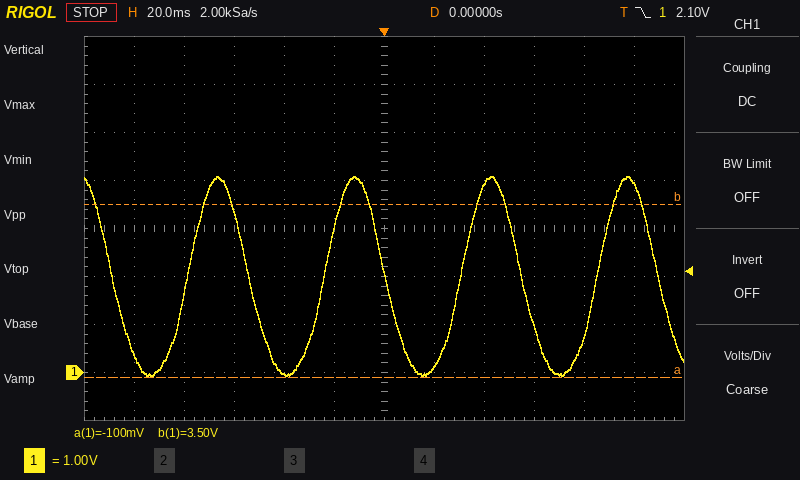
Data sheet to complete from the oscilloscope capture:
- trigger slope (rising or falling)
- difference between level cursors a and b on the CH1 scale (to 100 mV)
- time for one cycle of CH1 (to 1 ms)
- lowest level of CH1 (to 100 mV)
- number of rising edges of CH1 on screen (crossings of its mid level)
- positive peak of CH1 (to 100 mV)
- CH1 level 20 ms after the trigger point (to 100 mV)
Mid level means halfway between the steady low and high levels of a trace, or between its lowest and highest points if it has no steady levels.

falling
3.6 V
55 ms
-100 mV
4
4.1 V
100 mV
